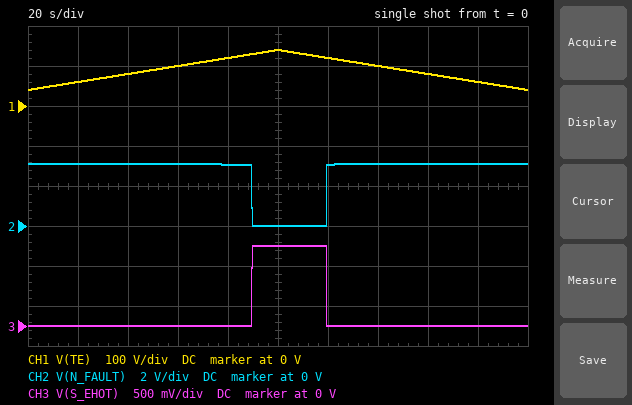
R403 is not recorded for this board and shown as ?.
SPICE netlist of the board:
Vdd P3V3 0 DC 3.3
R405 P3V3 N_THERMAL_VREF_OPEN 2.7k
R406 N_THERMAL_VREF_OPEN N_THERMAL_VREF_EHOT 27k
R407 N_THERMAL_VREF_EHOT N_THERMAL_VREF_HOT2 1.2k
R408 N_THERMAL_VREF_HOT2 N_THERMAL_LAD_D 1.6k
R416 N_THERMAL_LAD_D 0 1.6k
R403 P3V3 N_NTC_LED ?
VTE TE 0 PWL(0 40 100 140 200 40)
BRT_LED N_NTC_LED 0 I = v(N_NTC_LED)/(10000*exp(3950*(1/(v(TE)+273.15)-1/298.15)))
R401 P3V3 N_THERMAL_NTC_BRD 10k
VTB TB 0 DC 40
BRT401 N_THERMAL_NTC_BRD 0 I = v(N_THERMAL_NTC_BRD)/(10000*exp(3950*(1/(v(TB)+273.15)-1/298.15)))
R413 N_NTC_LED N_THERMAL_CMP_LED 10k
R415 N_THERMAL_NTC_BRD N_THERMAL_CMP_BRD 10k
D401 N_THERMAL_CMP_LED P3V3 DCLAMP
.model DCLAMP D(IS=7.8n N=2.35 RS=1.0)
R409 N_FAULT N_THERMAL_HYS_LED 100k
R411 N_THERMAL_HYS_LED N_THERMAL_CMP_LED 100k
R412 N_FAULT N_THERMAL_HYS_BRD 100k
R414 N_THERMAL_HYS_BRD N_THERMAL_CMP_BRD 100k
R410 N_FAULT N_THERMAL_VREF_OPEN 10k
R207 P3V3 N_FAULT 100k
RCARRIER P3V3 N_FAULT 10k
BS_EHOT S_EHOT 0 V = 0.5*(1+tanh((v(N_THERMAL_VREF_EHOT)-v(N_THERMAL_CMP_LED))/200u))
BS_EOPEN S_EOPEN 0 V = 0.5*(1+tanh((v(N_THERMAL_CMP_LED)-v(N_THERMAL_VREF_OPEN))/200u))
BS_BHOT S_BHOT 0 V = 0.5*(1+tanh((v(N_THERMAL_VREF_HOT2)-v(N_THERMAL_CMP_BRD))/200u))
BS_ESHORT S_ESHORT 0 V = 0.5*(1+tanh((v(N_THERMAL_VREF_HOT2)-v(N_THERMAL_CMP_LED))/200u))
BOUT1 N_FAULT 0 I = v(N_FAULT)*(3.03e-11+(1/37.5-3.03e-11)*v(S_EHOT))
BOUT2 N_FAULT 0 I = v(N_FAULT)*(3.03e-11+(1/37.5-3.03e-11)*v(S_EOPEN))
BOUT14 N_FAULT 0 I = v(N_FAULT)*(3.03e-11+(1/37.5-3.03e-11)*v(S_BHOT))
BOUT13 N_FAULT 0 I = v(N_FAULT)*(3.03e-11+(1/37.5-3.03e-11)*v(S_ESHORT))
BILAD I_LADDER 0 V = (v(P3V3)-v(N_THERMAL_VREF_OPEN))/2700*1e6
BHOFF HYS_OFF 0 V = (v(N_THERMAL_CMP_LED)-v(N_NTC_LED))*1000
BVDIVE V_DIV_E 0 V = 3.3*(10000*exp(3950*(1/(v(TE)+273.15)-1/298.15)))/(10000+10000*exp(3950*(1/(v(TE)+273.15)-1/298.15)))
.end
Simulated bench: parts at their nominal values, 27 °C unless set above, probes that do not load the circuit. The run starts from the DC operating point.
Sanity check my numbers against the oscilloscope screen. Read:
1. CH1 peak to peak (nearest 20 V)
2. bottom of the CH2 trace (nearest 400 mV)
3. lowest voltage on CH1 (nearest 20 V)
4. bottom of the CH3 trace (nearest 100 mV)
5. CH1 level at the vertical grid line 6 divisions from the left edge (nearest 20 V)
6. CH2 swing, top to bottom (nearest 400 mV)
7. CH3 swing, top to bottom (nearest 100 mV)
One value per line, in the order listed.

100 V
0 V
40 V
0 V
120 V
3.2 V
1.0 V
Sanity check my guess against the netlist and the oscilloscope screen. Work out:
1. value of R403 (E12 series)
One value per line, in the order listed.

3.3 kΩ
